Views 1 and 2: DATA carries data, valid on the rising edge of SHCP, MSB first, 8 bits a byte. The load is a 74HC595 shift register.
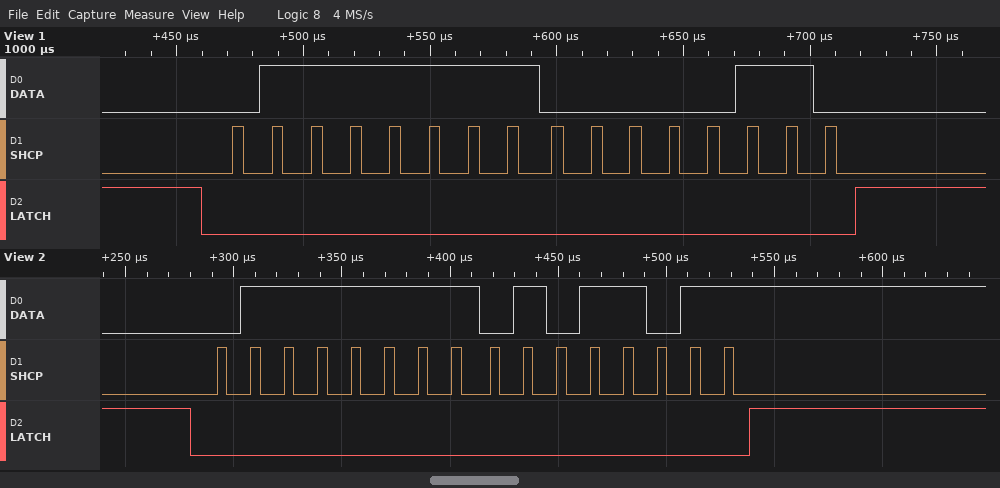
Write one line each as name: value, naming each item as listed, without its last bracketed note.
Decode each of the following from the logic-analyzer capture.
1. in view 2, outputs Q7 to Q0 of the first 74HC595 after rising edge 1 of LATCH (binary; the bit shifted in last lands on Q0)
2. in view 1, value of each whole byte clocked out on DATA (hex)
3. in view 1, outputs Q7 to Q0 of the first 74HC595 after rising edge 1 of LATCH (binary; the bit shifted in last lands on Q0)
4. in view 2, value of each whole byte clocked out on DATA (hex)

in view 2, outputs Q7 to Q0 of the first 74HC595 after rising edge 1 of LATCH: 01011011
in view 1, value of each whole byte clocked out on DATA: 0x7F 0x06
in view 1, outputs Q7 to Q0 of the first 74HC595 after rising edge 1 of LATCH: 00000110
in view 2, value of each whole byte clocked out on DATA: 7F 5B
